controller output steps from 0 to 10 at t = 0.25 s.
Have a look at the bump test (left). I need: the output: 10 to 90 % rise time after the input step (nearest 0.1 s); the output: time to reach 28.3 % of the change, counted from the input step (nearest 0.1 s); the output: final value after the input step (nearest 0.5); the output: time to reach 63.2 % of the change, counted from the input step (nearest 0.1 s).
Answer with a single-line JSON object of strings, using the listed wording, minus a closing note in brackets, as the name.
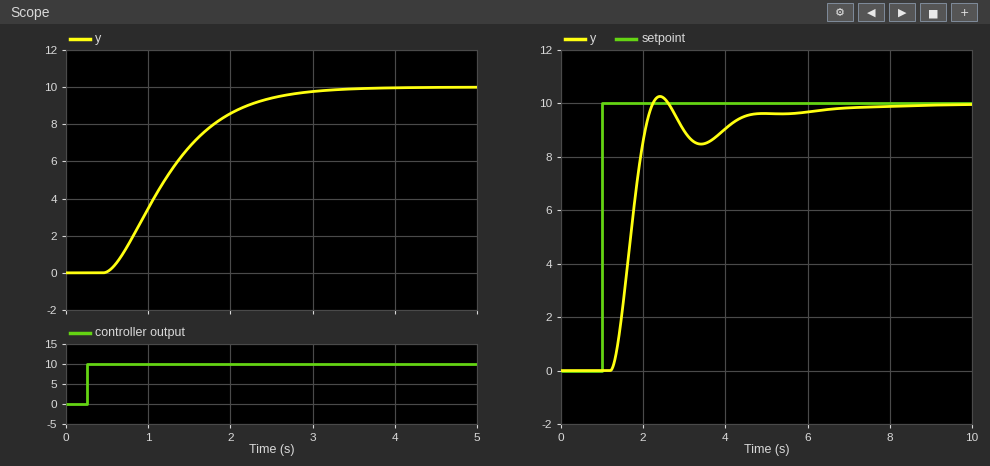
{"the output: 10 to 90 % rise time after the input step": "1.5 s", "the output: time to reach 28.3 % of the change, counted from the input step": "0.7 s", "the output: final value after the input step": "10.0", "the output: time to reach 63.2 % of the change, counted from the input step": "1.2 s"}
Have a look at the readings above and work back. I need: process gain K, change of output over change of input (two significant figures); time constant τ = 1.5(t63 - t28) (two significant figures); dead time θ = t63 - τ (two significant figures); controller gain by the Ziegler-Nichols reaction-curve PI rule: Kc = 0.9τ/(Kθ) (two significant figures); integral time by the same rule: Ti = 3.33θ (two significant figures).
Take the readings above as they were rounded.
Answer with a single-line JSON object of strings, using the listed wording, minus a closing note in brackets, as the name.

{"process gain K, change of output over change of input": "1.0", "time constant τ = 1.5(t63 - t28)": "0.75 s", "dead time θ = t63 - τ": "0.45 s", "controller gain by the Ziegler-Nichols reaction-curve PI rule: Kc = 0.9τ/(Kθ)": "1.5", "integral time by the same rule: Ti = 3.33θ": "1.5 s"}
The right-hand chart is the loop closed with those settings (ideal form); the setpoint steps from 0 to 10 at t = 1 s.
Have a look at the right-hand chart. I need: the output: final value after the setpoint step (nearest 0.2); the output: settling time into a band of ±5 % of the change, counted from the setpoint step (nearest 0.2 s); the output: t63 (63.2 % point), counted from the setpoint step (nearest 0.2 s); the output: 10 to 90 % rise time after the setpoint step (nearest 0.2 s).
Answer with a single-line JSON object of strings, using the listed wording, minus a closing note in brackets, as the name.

{"the output: final value after the setpoint step": "10.0", "the output: settling time into a band of ±5 % of the change, counted from the setpoint step": "3.4 s", "the output: t63 (63.2 % point), counted from the setpoint step": "0.8 s", "the output: 10 to 90 % rise time after the setpoint step": "0.6 s"}
